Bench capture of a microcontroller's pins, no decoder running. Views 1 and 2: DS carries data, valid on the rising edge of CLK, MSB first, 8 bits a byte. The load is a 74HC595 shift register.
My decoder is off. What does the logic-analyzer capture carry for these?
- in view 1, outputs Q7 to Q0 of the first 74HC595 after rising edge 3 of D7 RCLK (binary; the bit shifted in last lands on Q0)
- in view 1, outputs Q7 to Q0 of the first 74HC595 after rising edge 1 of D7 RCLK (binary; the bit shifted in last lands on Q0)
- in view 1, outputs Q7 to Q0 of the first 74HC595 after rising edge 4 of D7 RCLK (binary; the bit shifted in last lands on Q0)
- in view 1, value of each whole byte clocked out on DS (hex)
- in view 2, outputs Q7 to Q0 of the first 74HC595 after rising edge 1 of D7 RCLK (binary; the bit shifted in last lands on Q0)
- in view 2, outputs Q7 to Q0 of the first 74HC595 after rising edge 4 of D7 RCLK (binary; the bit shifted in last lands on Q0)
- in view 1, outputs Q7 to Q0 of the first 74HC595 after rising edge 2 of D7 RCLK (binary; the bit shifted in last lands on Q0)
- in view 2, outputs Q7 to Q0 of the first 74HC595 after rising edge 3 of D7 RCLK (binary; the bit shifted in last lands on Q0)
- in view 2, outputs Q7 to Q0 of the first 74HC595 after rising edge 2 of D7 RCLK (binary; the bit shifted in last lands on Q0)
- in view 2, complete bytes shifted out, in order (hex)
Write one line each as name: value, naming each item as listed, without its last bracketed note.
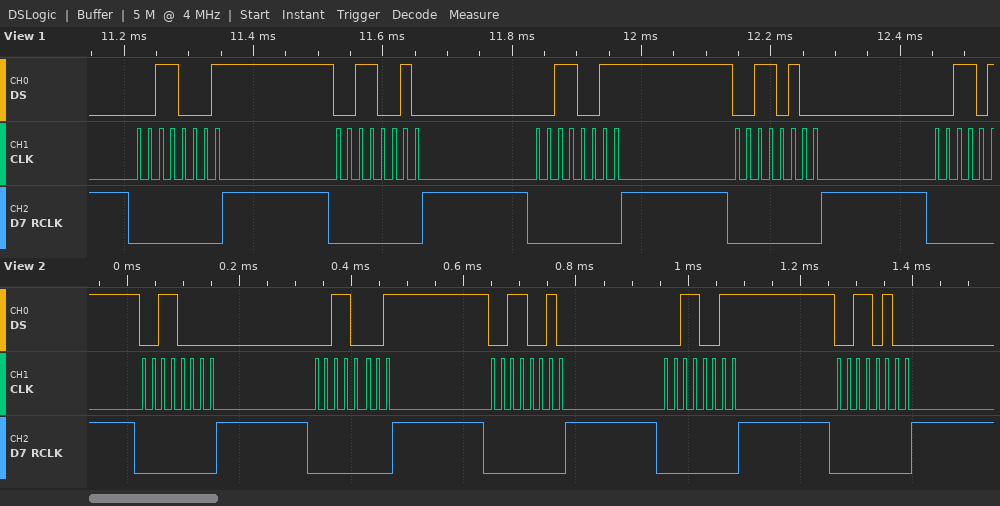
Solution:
in view 1, outputs Q7 to Q0 of the first 74HC595 after rising edge 3 of D7 RCLK: 00110011
in view 1, outputs Q7 to Q0 of the first 74HC595 after rising edge 1 of D7 RCLK: 00110001
in view 1, outputs Q7 to Q0 of the first 74HC595 after rising edge 4 of D7 RCLK: 00110100
in view 1, value of each whole byte clocked out on DS: 31 32 33 34
in view 2, outputs Q7 to Q0 of the first 74HC595 after rising edge 1 of D7 RCLK: 00110000
in view 2, outputs Q7 to Q0 of the first 74HC595 after rising edge 4 of D7 RCLK: 00110011
in view 1, outputs Q7 to Q0 of the first 74HC595 after rising edge 2 of D7 RCLK: 00110010
in view 2, outputs Q7 to Q0 of the first 74HC595 after rising edge 3 of D7 RCLK: 00110010
in view 2, outputs Q7 to Q0 of the first 74HC595 after rising edge 2 of D7 RCLK: 00110001
in view 2, complete bytes shifted out, in order: 30 31 32 33 34
